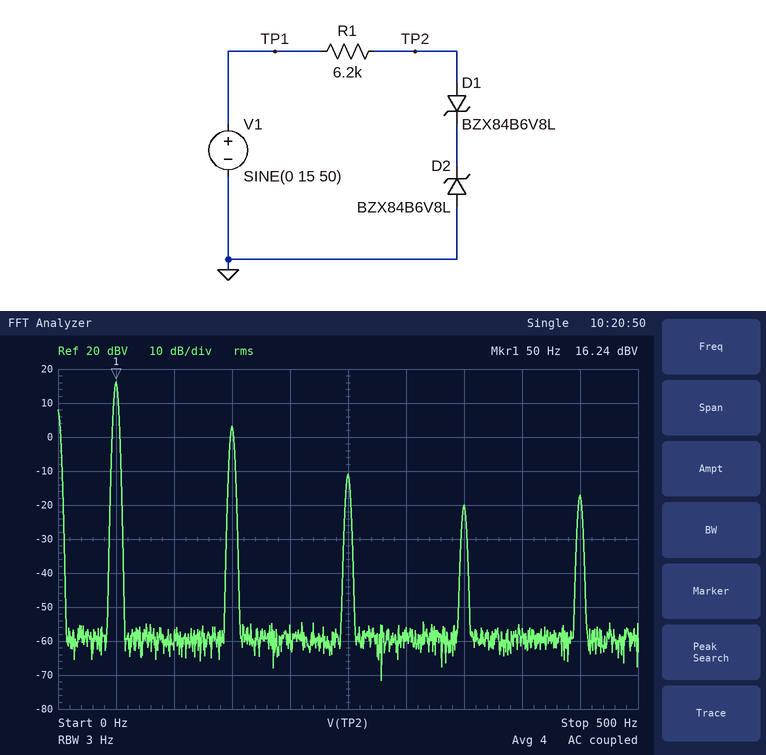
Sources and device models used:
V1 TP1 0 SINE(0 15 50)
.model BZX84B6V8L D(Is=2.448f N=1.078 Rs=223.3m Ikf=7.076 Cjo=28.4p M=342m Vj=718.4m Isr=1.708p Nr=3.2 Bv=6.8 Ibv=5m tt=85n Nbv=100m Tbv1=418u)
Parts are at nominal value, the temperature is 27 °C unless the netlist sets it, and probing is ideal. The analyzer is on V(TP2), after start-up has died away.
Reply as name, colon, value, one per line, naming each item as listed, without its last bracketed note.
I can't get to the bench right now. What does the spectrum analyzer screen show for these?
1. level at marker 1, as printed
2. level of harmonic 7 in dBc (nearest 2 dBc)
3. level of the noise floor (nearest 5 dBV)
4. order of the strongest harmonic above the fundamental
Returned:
level at marker 1, as printed: 16.24 dBV
level of harmonic 7 in dBc: -36 dBc
level of the noise floor: -60 dBV
order of the strongest harmonic above the fundamental: 3
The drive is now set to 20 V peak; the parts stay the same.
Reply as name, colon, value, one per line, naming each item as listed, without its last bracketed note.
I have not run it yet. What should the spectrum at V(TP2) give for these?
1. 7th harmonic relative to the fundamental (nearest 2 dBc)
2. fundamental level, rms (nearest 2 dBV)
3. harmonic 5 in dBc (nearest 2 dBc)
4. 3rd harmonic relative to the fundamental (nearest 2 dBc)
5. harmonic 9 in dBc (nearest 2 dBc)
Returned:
7th harmonic relative to the fundamental: -32 dBc
fundamental level, rms: 16 dBV
harmonic 5 in dBc: -20 dBc
3rd harmonic relative to the fundamental: -12 dBc
harmonic 9 in dBc: -42 dBc
